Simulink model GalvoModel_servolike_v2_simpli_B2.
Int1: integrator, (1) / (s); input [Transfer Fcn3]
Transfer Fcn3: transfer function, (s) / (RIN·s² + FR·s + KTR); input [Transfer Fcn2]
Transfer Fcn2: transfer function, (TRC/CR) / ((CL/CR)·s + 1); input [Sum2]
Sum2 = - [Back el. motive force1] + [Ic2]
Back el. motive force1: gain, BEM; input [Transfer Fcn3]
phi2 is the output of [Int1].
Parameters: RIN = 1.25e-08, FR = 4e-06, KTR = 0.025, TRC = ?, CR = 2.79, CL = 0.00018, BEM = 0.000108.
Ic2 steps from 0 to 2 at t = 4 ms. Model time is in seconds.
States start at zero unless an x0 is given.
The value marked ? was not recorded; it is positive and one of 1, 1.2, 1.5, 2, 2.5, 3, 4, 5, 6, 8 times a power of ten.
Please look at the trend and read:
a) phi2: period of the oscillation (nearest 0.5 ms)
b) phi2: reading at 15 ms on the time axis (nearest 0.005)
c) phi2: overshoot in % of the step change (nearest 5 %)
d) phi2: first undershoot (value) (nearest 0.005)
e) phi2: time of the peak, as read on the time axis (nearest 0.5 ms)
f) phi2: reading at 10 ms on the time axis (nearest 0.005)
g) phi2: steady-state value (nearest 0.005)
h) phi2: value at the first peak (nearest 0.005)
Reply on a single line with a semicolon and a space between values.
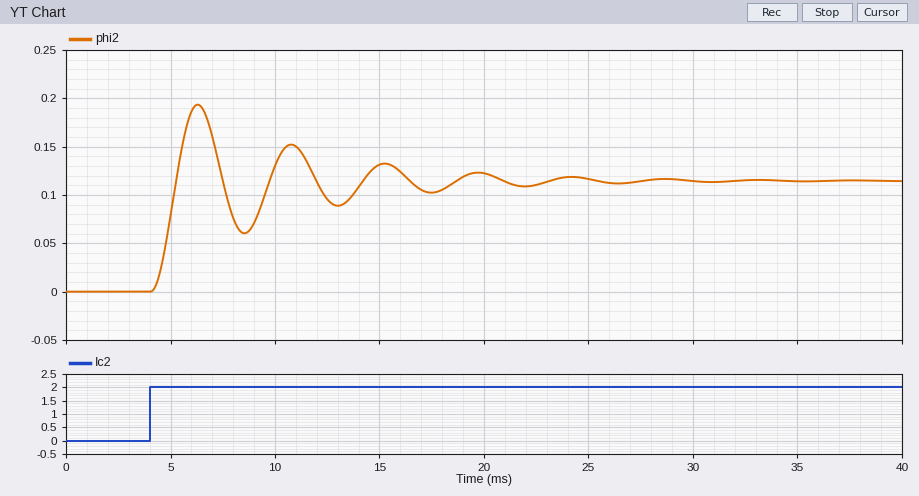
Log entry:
4.5 ms; 0.130; 70 %; 0.060; 6.5 ms; 0.130; 0.115; 0.195
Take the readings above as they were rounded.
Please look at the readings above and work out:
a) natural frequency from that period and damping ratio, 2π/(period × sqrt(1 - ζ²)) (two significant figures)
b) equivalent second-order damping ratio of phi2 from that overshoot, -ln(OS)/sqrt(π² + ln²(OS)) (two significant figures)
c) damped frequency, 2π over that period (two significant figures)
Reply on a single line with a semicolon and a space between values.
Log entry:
1.4 rad/ms; 0.11; 1.4 rad/ms
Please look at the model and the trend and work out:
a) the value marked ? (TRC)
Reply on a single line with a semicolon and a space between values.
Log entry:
0.004
